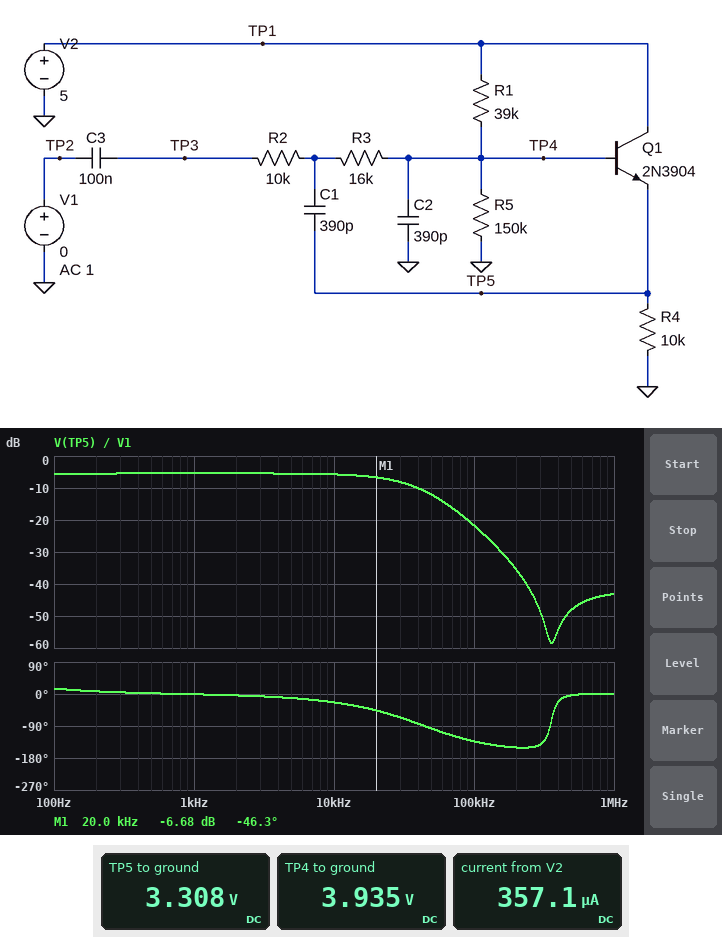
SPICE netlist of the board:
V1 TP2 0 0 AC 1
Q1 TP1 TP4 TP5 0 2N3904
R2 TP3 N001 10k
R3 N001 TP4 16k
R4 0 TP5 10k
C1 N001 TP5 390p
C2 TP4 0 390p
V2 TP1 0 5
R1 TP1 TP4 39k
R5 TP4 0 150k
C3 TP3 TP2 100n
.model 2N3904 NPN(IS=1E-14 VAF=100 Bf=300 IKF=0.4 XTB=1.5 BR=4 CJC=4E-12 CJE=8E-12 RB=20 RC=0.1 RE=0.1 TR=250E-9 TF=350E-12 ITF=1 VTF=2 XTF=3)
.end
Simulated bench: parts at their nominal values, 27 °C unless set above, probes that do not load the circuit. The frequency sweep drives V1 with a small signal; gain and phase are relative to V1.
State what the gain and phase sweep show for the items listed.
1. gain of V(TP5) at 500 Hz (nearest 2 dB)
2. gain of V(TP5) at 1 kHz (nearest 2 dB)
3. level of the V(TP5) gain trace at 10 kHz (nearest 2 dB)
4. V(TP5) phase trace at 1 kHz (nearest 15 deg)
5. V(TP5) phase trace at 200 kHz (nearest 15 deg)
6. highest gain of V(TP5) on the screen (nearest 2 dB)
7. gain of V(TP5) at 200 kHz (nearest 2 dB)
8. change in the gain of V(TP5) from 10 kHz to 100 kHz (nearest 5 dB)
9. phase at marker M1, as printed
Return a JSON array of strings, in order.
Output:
["-6 dB", "-6 dB", "-6 dB", "0 deg", "-150 deg", "-6 dB", "-36 dB", "-15 dB", "-46.3 deg"]
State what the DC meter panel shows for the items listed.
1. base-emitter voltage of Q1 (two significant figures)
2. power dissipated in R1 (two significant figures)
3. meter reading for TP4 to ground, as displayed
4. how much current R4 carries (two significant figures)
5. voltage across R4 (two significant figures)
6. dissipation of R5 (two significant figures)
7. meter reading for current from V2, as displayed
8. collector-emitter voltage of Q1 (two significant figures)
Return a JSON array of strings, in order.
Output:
["630 mV", "29 µW", "3.935 V", "330 µA", "3.3 V", "100 µW", "357.1 µA", "1.7 V"]
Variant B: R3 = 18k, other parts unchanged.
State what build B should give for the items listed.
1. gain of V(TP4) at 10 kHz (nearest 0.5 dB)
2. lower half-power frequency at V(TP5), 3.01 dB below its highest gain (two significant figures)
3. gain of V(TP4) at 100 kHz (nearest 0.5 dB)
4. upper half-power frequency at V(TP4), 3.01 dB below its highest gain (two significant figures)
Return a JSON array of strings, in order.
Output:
["-6.0 dB", "27 Hz", "-22.0 dB", "30 kHz"]
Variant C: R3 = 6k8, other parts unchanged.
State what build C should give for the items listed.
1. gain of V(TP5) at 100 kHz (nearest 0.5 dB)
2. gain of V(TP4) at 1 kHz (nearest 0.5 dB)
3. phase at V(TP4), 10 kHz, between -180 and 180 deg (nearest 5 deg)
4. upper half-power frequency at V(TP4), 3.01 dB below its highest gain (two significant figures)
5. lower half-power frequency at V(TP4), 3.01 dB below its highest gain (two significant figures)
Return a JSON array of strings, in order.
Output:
["-15.0 dB", "-4.0 dB", "-15 deg", "43 kHz", "33 Hz"]
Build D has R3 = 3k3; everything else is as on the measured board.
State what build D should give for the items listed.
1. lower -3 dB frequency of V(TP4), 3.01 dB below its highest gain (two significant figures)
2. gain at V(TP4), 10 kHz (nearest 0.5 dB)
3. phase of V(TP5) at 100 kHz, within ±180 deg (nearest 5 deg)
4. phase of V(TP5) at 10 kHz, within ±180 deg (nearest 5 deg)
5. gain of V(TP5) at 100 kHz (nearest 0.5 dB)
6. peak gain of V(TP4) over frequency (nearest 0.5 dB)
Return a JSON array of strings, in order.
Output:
["36 Hz", "-3.5 dB", "-100 deg", "-15 deg", "-11.5 dB", "-3.0 dB"]
